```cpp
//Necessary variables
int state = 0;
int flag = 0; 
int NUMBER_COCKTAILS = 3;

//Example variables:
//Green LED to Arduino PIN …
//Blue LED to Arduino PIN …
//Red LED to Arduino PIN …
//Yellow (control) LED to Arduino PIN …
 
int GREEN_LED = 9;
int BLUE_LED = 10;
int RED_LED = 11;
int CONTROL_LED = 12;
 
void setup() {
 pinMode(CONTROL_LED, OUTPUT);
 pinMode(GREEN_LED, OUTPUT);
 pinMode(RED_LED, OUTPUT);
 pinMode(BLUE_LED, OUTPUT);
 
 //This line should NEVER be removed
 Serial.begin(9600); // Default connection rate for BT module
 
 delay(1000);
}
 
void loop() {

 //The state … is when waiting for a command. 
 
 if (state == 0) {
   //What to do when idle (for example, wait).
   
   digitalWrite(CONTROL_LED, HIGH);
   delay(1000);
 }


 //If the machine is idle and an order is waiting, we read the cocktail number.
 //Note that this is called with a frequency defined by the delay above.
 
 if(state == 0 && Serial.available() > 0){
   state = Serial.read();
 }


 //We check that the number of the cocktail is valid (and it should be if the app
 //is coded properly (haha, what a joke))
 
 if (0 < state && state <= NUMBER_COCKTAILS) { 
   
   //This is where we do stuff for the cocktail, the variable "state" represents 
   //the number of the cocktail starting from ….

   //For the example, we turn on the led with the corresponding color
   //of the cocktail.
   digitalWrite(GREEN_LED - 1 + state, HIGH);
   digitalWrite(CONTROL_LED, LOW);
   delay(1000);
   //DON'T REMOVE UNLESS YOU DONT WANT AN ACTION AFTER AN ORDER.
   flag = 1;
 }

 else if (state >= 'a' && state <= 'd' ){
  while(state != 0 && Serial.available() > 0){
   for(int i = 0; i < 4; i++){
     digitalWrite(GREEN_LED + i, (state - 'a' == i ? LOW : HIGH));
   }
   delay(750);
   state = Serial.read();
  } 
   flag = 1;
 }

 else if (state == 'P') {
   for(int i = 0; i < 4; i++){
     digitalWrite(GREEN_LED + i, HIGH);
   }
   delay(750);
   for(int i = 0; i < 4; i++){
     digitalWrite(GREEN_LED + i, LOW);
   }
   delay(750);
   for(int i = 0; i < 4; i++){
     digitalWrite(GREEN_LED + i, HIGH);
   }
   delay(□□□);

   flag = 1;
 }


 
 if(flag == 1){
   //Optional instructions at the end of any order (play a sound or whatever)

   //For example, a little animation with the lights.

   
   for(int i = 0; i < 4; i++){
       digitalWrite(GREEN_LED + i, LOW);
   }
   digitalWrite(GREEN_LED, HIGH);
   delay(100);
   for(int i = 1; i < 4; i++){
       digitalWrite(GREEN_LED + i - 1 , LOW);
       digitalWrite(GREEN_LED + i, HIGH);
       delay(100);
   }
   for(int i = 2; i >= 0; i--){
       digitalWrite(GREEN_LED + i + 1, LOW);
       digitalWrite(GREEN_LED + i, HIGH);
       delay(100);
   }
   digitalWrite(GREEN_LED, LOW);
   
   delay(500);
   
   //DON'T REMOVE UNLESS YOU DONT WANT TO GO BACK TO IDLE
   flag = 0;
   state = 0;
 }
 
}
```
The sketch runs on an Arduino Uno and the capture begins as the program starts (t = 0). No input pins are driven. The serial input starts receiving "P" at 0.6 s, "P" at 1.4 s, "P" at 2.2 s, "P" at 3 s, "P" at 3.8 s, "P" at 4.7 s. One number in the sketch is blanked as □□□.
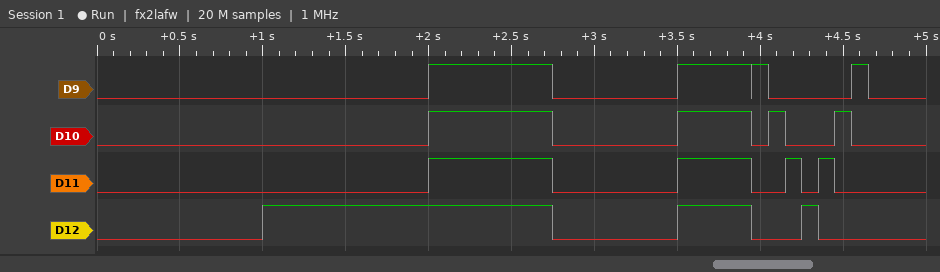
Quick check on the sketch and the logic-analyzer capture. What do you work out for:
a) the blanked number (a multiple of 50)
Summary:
450
